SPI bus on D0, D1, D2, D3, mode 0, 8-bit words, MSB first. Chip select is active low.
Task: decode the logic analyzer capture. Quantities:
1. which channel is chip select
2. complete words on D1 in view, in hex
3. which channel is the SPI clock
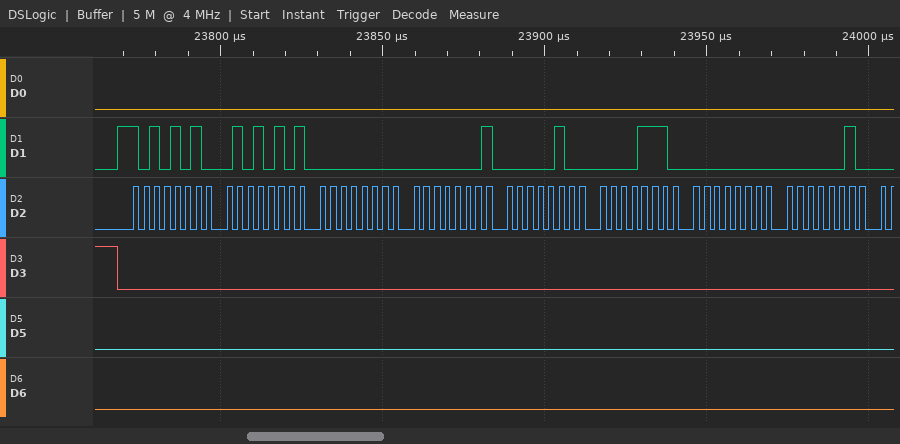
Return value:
D3
AA, 55, 00, 01, 04, 0E, 00, 02
D2
